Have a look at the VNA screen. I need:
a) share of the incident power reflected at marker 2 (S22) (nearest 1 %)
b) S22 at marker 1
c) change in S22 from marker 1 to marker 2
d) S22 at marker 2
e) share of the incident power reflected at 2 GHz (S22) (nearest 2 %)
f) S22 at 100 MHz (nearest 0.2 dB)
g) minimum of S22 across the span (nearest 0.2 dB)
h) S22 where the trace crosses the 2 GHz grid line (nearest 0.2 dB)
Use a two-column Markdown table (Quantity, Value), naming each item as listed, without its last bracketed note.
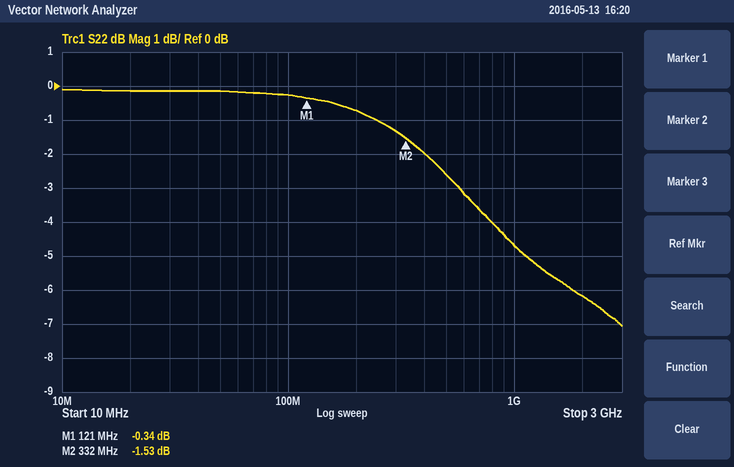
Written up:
| Quantity | Value |
|---|---|
| share of the incident power reflected at marker 2 (S22) | 70 % |
| S22 at marker 1 | -0.34 dB |
| change in S22 from marker 1 to marker 2 | -1.19 dB |
| S22 at marker 2 | -1.53 dB |
| share of the incident power reflected at 2 GHz (S22) | 24 % |
| S22 at 100 MHz | -0.2 dB |
| minimum of S22 across the span | -7.0 dB |
| S22 where the trace crosses the 2 GHz grid line | -6.2 dB |
